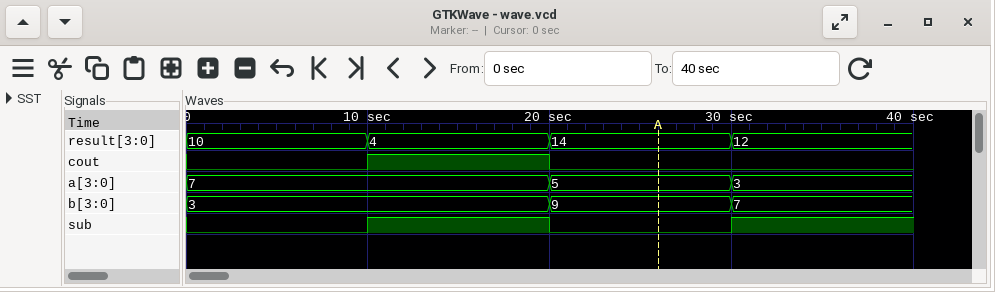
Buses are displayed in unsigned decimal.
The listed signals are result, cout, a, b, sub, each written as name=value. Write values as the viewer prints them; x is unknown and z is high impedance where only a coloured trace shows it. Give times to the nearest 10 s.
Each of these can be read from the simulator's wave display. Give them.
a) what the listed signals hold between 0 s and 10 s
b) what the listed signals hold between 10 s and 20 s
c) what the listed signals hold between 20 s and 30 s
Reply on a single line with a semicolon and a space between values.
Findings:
result=10, cout=0, a=7, b=3, sub=0; result=4, cout=1, a=7, b=3, sub=1; result=14, cout=0, a=5, b=9, sub=0
